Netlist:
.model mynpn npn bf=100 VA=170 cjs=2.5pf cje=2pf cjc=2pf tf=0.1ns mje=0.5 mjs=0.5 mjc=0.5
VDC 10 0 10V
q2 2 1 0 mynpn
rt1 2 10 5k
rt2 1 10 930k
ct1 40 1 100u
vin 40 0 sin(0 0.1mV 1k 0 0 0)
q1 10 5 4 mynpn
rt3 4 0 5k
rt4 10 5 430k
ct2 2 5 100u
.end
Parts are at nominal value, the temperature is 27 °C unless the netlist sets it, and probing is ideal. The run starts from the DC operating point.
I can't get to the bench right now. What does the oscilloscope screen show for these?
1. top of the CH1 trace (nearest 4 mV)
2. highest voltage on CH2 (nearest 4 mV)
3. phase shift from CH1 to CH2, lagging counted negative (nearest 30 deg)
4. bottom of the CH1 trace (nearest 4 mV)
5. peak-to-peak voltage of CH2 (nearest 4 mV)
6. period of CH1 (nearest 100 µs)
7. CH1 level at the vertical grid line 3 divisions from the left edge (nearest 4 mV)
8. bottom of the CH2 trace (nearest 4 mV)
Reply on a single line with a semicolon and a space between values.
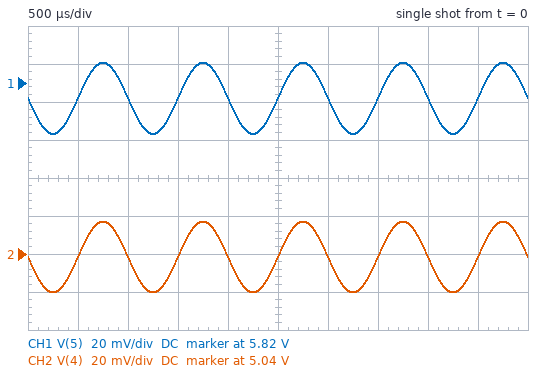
5.832 V; 5.056 V; 0 deg; 5.792 V; 36 mV; 1.0 ms; 5.812 V; 5.020 V
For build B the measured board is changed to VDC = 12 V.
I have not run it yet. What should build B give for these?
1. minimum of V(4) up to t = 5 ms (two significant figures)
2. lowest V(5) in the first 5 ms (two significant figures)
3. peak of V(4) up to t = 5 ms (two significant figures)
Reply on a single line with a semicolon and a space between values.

6.1 V; 6.9 V; 6.2 V
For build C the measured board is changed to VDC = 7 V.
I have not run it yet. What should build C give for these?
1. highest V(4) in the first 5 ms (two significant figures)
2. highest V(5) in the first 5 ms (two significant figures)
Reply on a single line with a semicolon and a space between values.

3.4 V; 4.2 V
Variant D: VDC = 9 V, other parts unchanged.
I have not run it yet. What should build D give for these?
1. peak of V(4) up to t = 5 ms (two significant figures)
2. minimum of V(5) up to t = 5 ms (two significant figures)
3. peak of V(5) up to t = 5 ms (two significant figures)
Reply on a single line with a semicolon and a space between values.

4.5 V; 5.2 V; 5.3 V
